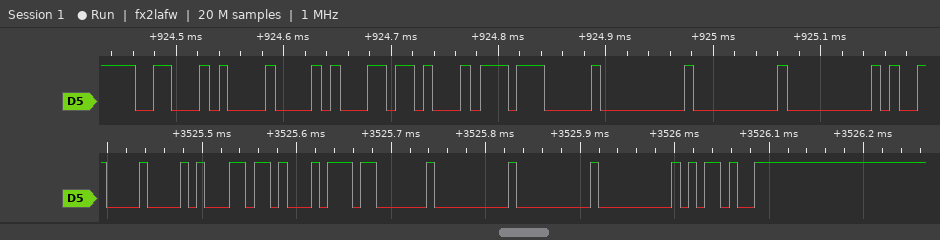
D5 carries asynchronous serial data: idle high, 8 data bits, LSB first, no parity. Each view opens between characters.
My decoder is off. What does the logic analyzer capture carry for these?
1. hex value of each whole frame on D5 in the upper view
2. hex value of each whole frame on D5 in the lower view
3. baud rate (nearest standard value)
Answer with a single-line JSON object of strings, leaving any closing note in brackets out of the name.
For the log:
{"hex value of each whole frame on D5 in the upper view": "46, 08, B1, D1, 07, 00, 00, 00", "hex value of each whole frame on D5 in the lower view": "08, B1, D1, 03, 00, 00, 00, 2D", "baud rate": "115200 baud"}
